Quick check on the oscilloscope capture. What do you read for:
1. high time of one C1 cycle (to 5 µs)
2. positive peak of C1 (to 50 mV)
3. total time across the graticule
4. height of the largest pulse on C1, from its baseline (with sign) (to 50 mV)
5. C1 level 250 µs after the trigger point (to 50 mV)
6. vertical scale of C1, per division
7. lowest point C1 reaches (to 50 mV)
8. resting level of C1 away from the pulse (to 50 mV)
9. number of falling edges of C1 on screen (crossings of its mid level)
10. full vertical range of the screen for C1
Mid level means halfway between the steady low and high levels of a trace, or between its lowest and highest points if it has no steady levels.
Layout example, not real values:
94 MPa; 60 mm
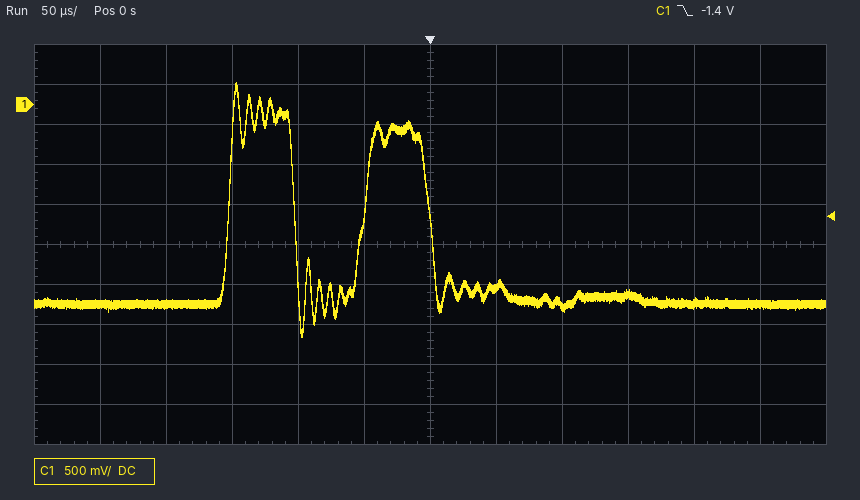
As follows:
50 µs; 250 mV; 600 µs; +2.75 V; -2.50 V; 500 mV; -2.90 V; -2.50 V; 2; 5 V
